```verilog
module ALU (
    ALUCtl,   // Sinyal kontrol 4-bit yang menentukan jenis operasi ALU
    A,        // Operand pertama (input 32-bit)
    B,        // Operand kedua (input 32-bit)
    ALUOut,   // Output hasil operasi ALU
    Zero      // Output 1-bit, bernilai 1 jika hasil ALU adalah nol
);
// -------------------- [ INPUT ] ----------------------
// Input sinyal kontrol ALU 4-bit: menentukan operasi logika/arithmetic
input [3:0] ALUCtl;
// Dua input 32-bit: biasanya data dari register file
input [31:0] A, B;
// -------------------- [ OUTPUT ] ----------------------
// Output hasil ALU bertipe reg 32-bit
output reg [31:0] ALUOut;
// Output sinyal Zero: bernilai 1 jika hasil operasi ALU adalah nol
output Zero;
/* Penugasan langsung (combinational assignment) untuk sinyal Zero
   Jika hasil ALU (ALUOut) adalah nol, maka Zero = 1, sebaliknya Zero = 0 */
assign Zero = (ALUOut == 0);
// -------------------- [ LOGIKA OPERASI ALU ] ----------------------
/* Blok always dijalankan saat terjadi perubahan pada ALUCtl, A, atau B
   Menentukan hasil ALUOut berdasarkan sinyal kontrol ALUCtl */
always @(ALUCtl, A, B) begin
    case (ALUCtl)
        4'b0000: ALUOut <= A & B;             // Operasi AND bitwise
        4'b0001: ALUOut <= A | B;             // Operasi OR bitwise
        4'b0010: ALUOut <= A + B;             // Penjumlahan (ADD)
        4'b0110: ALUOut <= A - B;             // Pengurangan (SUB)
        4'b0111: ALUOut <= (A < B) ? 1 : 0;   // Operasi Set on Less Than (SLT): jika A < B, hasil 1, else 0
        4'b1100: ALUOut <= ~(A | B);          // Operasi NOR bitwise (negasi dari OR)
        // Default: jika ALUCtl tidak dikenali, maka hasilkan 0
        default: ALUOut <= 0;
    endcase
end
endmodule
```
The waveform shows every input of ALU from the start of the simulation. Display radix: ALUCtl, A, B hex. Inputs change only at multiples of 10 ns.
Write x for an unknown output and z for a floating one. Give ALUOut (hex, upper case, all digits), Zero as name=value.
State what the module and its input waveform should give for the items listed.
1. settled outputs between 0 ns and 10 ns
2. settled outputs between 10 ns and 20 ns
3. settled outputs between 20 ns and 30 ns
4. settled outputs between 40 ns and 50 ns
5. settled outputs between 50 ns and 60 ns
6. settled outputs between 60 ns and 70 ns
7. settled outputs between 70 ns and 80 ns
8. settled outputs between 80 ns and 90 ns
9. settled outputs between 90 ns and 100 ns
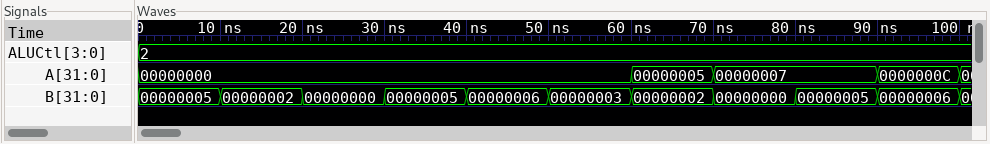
ALUOut=00000005, Zero=0
ALUOut=00000002, Zero=0
ALUOut=00000000, Zero=1
ALUOut=00000006, Zero=0
ALUOut=00000003, Zero=0
ALUOut=00000007, Zero=0
ALUOut=00000007, Zero=0
ALUOut=0000000C, Zero=0
ALUOut=00000012, Zero=0
